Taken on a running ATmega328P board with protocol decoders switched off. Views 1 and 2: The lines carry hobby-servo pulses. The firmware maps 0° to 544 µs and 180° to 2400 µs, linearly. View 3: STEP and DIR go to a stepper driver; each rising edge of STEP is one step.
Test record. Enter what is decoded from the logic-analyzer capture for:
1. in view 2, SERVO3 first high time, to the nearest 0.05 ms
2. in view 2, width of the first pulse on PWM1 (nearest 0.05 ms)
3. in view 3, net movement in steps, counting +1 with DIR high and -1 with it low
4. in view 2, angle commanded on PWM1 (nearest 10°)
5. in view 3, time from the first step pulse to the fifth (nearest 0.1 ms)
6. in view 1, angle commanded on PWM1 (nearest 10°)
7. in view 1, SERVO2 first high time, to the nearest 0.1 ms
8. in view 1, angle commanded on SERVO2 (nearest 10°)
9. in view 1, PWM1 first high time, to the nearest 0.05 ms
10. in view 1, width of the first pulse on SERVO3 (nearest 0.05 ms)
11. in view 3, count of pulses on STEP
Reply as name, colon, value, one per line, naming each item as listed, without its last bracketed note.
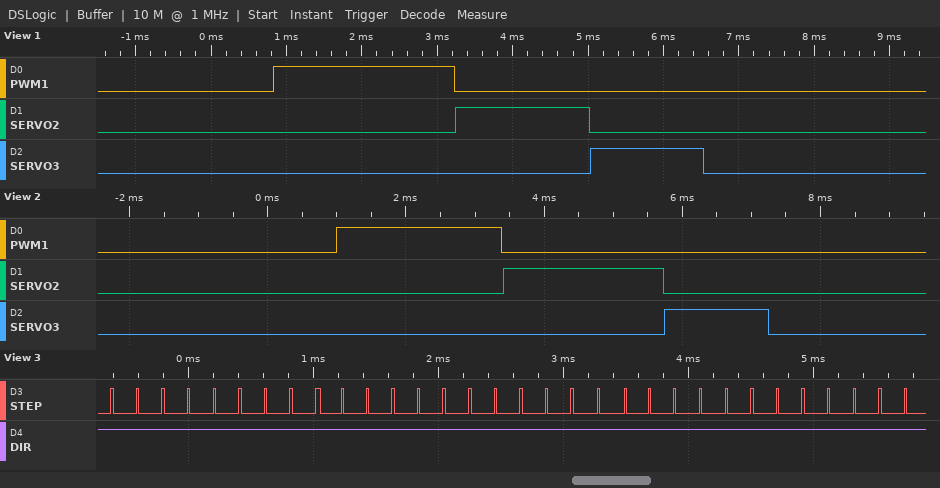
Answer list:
in view 2, SERVO3 first high time, to the nearest 0.05 ms: 1.50 ms
in view 2, width of the first pulse on PWM1: 2.40 ms
in view 3, net movement in steps, counting +1 with DIR high and -1 with it low: +32
in view 2, angle commanded on PWM1: 180°
in view 3, time from the first step pulse to the fifth: 0.8 ms
in view 1, angle commanded on PWM1: 180°
in view 1, SERVO2 first high time, to the nearest 0.1 ms: 1.8 ms
in view 1, angle commanded on SERVO2: 120°
in view 1, PWM1 first high time, to the nearest 0.05 ms: 2.40 ms
in view 1, width of the first pulse on SERVO3: 1.50 ms
in view 3, count of pulses on STEP: 32
